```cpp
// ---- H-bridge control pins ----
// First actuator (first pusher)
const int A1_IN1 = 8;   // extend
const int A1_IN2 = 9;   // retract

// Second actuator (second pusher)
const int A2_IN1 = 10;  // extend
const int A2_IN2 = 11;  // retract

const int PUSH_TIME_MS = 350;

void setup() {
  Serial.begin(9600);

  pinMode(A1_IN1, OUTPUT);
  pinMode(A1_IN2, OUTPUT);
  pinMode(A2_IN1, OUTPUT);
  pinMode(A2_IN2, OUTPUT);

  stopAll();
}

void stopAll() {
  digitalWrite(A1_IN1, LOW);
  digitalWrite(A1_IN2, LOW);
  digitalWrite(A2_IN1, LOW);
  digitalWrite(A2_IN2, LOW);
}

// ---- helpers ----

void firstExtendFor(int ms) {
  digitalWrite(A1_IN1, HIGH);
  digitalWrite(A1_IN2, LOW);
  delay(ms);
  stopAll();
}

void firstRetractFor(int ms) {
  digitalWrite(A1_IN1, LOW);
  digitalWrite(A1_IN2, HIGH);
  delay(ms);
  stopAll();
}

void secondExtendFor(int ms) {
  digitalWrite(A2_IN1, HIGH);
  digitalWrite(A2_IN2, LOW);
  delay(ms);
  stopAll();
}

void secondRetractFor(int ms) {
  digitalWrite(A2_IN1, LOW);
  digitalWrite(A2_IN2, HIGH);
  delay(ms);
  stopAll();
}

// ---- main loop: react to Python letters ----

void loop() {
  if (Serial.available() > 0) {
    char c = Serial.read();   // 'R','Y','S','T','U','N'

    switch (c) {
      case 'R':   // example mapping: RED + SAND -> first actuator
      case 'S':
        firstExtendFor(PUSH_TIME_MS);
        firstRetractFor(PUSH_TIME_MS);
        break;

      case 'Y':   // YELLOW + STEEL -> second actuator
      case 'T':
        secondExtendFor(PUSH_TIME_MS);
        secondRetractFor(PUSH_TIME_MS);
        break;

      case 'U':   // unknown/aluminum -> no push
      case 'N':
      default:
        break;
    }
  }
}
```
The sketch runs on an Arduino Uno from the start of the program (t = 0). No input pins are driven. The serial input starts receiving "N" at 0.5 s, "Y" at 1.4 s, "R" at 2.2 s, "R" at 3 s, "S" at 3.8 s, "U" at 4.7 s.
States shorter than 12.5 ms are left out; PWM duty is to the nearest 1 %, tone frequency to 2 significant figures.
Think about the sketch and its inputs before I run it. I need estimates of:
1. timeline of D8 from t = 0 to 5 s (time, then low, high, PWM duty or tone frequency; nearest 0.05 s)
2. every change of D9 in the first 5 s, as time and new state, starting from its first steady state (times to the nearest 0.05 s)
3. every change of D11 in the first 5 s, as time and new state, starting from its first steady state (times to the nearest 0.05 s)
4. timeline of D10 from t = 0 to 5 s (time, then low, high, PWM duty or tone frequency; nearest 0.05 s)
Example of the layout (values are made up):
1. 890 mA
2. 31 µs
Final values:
1. 0 s low; 2.2 s high; 2.55 s low; 3 s high; 3.35 s low; 3.8 s high; 4.15 s low
2. 0 s low; 2.55 s high; 2.9 s low; 3.35 s high; 3.7 s low; 4.15 s high; 4.5 s low
3. 0 s low; 1.75 s high; 2.1 s low
4. 0 s low; 1.4 s high; 1.75 s low
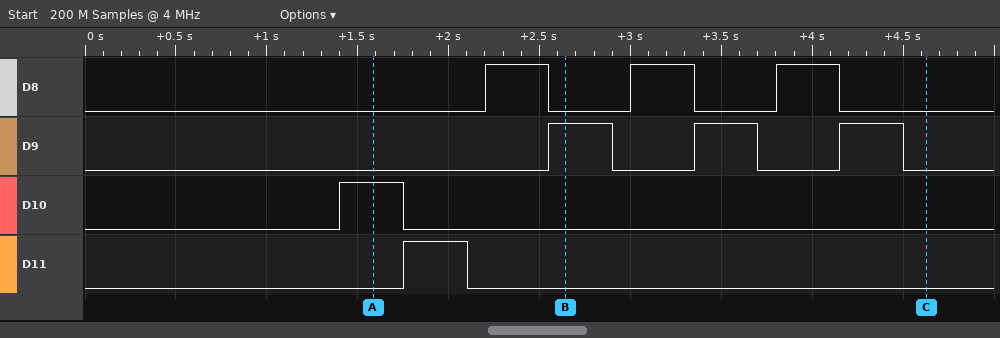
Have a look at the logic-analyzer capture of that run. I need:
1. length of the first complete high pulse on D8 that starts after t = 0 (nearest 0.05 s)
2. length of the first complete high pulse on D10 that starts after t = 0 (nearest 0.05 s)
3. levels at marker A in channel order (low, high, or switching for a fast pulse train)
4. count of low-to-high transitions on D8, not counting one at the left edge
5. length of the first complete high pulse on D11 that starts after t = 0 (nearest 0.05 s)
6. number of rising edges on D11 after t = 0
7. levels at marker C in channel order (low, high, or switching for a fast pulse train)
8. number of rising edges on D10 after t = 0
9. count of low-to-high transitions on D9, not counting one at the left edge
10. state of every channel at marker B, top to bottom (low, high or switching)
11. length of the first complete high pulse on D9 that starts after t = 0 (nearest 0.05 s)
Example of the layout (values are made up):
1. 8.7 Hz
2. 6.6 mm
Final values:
1. 0.35 s
2. 0.35 s
3. D8 low, D9 low, D10 high, D11 low
4. 3
5. 0.35 s
6. 1
7. D8 low, D9 low, D10 low, D11 low
8. 1
9. 3
10. D8 low, D9 high, D10 low, D11 low
11. 0.35 s
